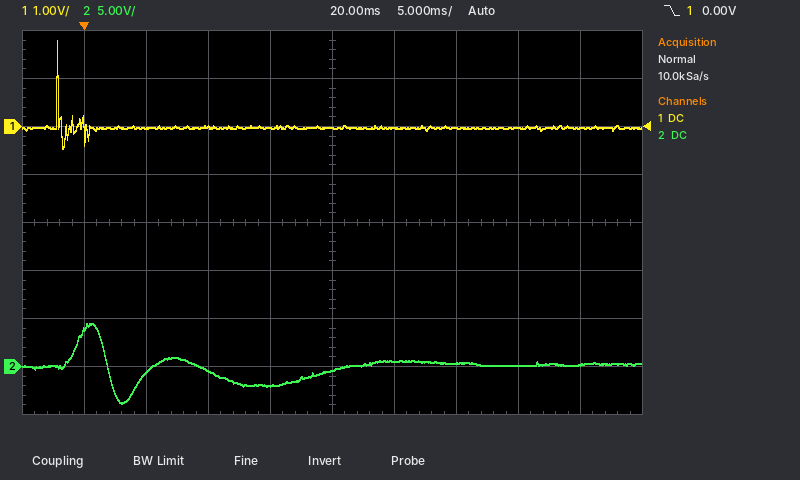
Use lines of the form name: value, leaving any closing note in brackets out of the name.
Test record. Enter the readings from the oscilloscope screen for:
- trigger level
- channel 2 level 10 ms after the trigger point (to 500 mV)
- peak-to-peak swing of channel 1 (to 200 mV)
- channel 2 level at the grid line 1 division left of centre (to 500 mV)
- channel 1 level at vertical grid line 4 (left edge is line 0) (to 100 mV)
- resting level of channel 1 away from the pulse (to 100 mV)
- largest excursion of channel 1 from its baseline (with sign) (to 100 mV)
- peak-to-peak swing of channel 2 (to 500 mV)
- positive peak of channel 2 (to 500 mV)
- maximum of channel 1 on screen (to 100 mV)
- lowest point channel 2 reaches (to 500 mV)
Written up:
trigger level: 0.00 V
channel 2 level 10 ms after the trigger point: -500 mV
peak-to-peak swing of channel 1: 2.2 V
channel 2 level at the grid line 1 division left of centre: -2.0 V
channel 1 level at vertical grid line 4 (left edge is line 0): 0.0 V
resting level of channel 1 away from the pulse: 0.0 V
largest excursion of channel 1 from its baseline (with sign): +1.8 V
peak-to-peak swing of channel 2: 8.5 V
positive peak of channel 2: 4.5 V
maximum of channel 1 on screen: 1.8 V
lowest point channel 2 reaches: -4.0 V
